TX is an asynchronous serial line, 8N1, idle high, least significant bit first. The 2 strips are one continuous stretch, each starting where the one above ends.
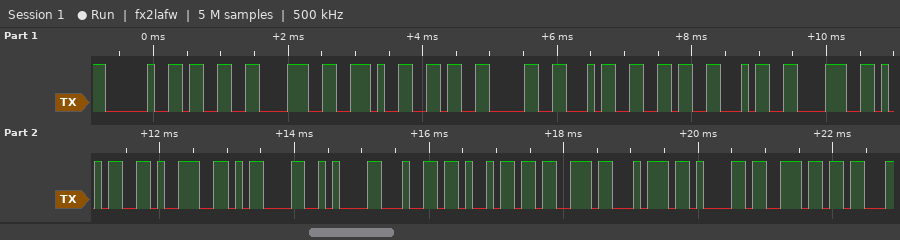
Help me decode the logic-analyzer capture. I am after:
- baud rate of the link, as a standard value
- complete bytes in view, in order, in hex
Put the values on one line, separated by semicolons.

9600 baud; 0x20 0x33 0x38 0x2E 0x36 0x30 0x34 0x36 0x34 0x38 0x35 0x39 0x0D 0x0A 0x64 0x69 0x73 0x74 0x61 0x6E
